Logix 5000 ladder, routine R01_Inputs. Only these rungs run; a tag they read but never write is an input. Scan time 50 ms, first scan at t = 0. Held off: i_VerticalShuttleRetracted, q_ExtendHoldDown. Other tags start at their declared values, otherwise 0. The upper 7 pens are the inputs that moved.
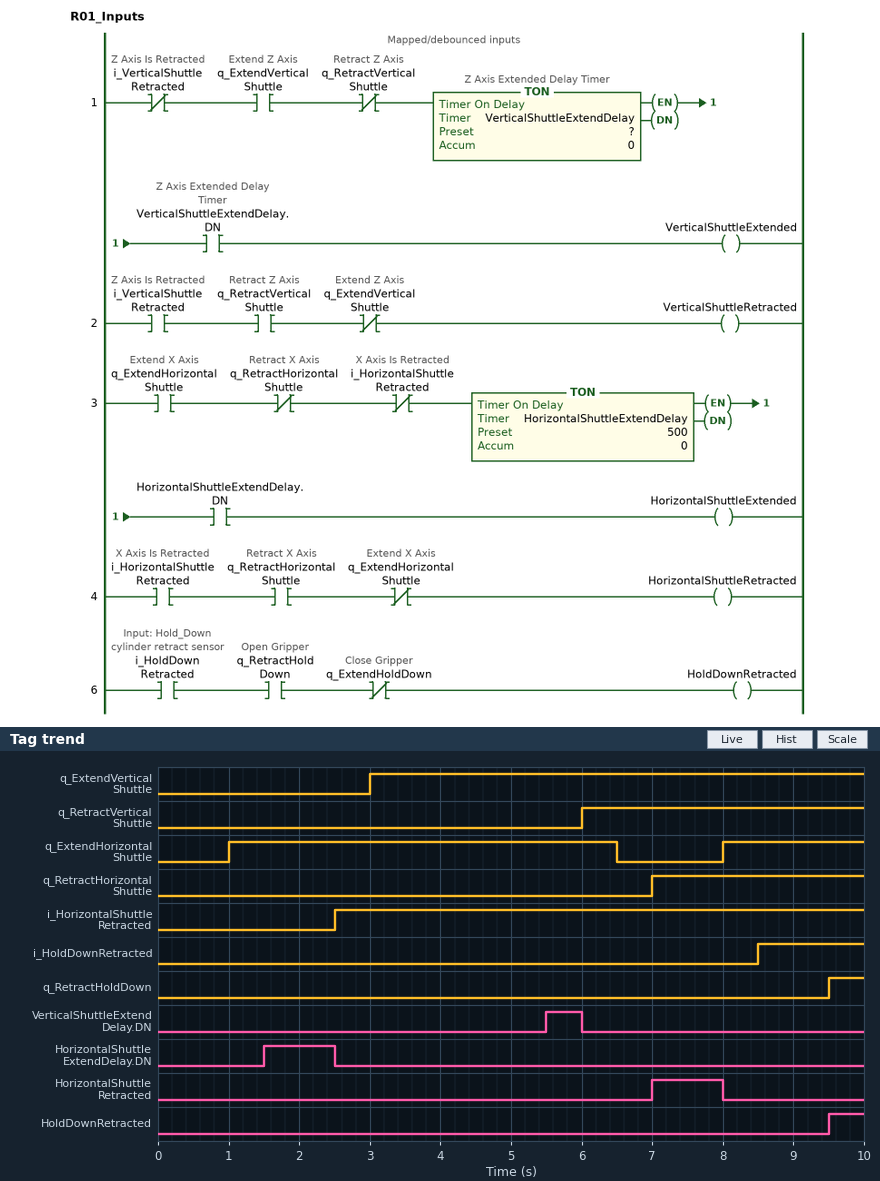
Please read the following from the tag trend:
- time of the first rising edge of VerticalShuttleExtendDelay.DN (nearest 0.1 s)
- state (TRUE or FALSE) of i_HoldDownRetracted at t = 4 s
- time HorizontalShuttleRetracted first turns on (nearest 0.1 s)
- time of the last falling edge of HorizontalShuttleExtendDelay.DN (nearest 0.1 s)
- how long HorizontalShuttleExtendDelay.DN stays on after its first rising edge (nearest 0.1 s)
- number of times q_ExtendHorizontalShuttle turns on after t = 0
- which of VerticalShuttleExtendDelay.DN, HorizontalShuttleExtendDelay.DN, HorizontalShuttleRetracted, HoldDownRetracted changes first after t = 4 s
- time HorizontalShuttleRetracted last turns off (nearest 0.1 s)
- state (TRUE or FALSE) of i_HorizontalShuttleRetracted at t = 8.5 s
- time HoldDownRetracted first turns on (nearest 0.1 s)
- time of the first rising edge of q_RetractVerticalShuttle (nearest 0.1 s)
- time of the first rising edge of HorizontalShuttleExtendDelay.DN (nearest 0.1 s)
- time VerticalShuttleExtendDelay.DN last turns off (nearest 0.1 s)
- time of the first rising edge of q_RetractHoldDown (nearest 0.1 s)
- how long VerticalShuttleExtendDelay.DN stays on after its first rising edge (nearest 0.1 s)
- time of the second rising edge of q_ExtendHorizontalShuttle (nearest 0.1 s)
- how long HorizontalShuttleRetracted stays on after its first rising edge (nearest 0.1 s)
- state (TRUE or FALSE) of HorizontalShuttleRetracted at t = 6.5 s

5.5 s
FALSE
7.0 s
2.5 s
1.0 s
2
VerticalShuttleExtendDelay.DN
8.0 s
TRUE
9.5 s
6.0 s
1.5 s
6.0 s
9.5 s
0.5 s
8.0 s
1.0 s
FALSE
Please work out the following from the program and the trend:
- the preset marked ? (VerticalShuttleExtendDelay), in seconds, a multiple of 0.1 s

2.5 s
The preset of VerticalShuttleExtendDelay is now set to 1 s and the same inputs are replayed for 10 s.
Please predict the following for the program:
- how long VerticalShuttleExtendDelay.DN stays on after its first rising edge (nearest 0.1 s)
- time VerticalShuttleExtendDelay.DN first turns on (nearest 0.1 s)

2.0 s
4.0 s
